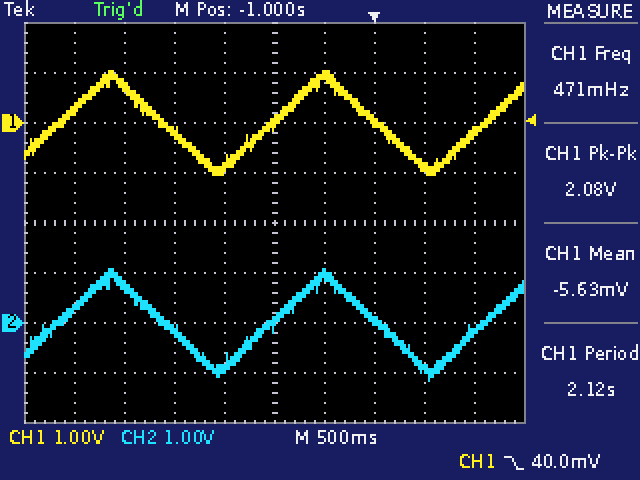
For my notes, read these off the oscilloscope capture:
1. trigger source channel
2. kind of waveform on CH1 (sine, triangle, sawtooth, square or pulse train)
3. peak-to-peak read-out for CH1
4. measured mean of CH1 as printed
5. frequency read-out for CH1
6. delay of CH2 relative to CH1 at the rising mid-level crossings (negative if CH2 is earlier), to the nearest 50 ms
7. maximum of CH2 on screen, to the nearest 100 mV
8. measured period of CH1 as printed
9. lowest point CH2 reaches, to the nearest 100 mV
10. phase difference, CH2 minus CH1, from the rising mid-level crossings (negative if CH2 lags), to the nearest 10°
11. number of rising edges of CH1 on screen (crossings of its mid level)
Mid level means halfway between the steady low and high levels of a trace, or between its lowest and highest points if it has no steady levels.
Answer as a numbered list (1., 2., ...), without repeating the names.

1. CH1
2. triangle
3. 2.08 V
4. -5.63 mV
5. 471 mHz
6. -50 ms
7. 1.1 V
8. 2.12 s
9. -1.2 V
10. +10°
11. 3
